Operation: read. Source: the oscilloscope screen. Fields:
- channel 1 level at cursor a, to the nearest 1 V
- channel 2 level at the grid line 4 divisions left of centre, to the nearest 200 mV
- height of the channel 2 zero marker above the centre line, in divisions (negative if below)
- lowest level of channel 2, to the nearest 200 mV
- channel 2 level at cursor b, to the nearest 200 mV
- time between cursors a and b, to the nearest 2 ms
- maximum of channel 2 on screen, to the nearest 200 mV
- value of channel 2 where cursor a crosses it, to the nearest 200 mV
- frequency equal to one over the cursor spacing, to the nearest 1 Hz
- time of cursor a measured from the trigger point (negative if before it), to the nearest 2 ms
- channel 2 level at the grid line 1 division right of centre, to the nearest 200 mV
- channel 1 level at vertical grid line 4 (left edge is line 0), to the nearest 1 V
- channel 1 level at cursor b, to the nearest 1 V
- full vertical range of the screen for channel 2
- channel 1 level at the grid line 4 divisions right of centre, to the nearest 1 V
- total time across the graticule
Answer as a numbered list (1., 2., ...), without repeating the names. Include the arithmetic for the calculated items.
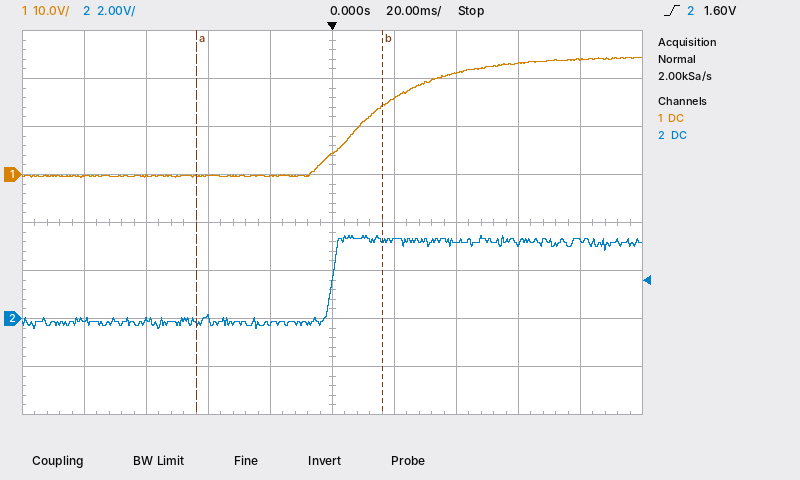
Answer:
1. 0 V
2. 0.0 V
3. -2.0 div
4. -400 mV
5. 3.2 V
6. 60 ms
7. 3.4 V
8. -200 mV
9. 1 / 60 ms ≈ 17 Hz
10. -44 ms
11. 3.2 V
12. 0 V
13. 14 V
14. 16 V
15. 24 V
16. 200 ms
